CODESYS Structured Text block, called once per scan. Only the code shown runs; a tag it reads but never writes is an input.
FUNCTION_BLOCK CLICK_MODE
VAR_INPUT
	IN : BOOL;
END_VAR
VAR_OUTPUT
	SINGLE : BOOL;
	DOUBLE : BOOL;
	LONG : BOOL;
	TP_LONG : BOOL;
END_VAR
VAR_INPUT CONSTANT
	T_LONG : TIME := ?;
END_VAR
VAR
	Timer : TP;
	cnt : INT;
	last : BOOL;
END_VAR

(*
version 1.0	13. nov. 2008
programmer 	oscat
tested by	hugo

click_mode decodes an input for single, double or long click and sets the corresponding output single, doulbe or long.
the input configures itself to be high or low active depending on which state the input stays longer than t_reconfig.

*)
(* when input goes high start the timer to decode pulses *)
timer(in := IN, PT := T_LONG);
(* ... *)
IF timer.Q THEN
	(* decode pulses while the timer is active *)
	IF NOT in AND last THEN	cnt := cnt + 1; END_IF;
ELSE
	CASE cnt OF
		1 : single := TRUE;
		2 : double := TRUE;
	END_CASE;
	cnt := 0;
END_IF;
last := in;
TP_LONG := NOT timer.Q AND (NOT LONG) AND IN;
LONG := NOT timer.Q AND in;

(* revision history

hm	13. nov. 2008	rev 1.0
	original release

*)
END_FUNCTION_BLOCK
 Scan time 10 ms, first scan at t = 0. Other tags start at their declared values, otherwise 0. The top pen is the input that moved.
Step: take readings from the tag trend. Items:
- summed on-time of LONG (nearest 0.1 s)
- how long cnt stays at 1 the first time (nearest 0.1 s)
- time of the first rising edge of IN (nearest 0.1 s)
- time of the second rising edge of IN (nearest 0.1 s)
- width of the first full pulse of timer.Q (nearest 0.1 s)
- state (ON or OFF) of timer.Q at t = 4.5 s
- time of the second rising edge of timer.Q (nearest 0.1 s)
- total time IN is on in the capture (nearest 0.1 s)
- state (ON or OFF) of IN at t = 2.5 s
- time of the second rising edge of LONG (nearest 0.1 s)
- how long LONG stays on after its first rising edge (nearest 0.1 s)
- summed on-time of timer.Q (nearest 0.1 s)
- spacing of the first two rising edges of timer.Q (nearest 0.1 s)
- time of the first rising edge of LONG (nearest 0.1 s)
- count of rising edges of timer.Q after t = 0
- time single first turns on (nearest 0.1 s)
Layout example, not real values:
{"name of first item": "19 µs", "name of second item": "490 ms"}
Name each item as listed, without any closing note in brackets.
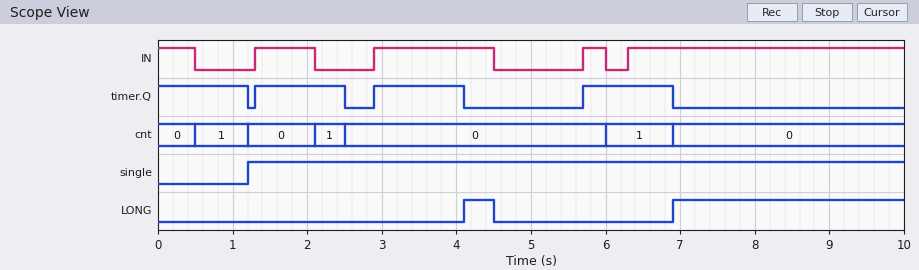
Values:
{"summed on-time of LONG": "3.5 s", "how long cnt stays at 1 the first time": "0.7 s", "time of the first rising edge of IN": "1.3 s", "time of the second rising edge of IN": "2.9 s", "width of the first full pulse of timer.Q": "1.2 s", "state (ON or OFF) of timer.Q at t = 4.5 s": "OFF", "time of the second rising edge of timer.Q": "2.9 s", "total time IN is on in the capture": "6.9 s", "state (ON or OFF) of IN at t = 2.5 s": "OFF", "time of the second rising edge of LONG": "6.9 s", "how long LONG stays on after its first rising edge": "0.4 s", "summed on-time of timer.Q": "4.8 s", "spacing of the first two rising edges of timer.Q": "1.6 s", "time of the first rising edge of LONG": "4.1 s", "count of rising edges of timer.Q after t = 0": "3", "time single first turns on": "1.2 s"}
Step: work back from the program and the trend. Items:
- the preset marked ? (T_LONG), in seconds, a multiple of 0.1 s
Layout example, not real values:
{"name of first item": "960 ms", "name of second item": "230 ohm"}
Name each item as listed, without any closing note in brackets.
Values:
{"the preset marked ? (T_LONG), in seconds, a multiple of 0.1 s": "1.2 s"}
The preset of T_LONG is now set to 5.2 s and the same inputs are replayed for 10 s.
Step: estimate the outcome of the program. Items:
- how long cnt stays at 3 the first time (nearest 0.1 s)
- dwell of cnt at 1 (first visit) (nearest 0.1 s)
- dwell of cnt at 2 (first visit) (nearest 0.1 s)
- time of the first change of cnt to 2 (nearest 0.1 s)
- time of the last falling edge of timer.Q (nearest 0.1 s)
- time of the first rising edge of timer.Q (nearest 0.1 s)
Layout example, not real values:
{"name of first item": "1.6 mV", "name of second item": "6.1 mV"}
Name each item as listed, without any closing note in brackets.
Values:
{"how long cnt stays at 3 the first time": "0.7 s", "dwell of cnt at 1 (first visit)": "1.6 s", "dwell of cnt at 2 (first visit)": "2.4 s", "time of the first change of cnt to 2": "2.1 s", "time of the last falling edge of timer.Q": "5.2 s", "time of the first rising edge of timer.Q": "5.7 s"}
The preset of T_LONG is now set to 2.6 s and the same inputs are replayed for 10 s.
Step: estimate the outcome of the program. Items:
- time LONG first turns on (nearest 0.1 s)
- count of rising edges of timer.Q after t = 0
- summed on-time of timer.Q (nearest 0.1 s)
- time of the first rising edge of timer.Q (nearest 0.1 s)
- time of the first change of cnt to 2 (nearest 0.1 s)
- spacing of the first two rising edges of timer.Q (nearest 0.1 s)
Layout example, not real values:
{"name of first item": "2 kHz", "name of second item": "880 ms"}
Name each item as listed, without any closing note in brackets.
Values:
{"time LONG first turns on": "8.3 s", "count of rising edges of timer.Q after t = 0": "2", "summed on-time of timer.Q": "7.8 s", "time of the first rising edge of timer.Q": "2.9 s", "time of the first change of cnt to 2": "2.1 s", "spacing of the first two rising edges of timer.Q": "2.8 s"}
